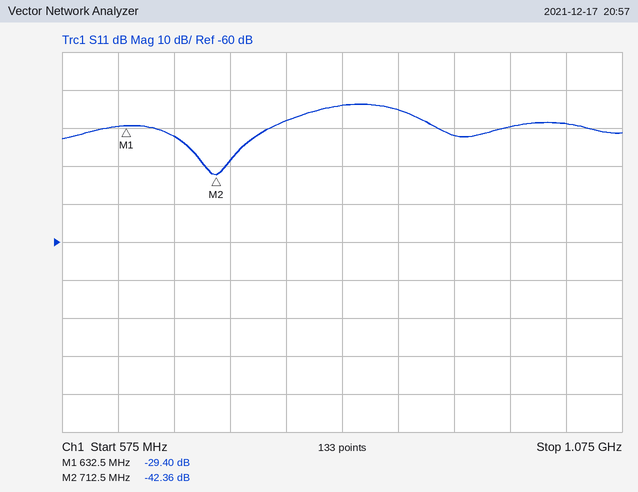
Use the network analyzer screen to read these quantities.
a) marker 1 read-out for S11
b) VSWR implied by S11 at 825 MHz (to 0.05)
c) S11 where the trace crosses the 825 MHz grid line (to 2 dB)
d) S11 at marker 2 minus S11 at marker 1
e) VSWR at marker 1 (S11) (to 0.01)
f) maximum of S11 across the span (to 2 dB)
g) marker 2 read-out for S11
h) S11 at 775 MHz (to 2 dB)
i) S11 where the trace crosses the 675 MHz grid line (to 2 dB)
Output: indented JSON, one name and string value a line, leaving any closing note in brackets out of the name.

{
  "marker 1 read-out for S11": "-29.40 dB",
  "VSWR implied by S11 at 825 MHz": "1.15",
  "S11 where the trace crosses the 825 MHz grid line": "-24 dB",
  "S11 at marker 2 minus S11 at marker 1": "-12.96 dB",
  "VSWR at marker 1 (S11)": "1.07",
  "maximum of S11 across the span": "-24 dB",
  "marker 2 read-out for S11": "-42.36 dB",
  "S11 at 775 MHz": "-28 dB",
  "S11 where the trace crosses the 675 MHz grid line": "-32 dB"
}
